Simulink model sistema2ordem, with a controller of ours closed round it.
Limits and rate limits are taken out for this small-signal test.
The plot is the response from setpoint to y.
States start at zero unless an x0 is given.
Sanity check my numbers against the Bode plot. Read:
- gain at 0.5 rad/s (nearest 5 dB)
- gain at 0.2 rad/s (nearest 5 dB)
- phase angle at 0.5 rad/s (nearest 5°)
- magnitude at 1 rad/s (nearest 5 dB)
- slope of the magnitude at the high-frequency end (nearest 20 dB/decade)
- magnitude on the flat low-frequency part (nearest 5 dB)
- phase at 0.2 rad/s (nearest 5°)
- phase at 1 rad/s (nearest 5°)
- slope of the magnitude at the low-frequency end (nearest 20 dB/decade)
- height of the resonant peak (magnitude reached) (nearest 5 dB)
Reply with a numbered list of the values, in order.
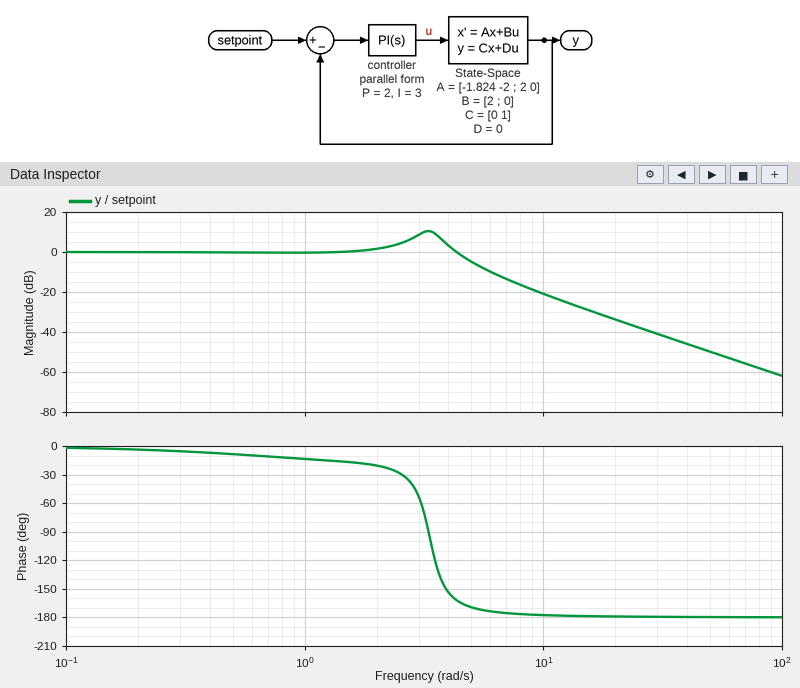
1. 0 dB
2. 0 dB
3. -10°
4. 0 dB
5. -40 dB/decade
6. 0 dB
7. -5°
8. -15°
9. 0 dB/decade
10. 10 dB
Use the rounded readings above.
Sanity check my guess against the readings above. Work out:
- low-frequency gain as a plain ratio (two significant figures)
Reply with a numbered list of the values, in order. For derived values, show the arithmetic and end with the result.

1. 10^(0 / 20) = 1.0
